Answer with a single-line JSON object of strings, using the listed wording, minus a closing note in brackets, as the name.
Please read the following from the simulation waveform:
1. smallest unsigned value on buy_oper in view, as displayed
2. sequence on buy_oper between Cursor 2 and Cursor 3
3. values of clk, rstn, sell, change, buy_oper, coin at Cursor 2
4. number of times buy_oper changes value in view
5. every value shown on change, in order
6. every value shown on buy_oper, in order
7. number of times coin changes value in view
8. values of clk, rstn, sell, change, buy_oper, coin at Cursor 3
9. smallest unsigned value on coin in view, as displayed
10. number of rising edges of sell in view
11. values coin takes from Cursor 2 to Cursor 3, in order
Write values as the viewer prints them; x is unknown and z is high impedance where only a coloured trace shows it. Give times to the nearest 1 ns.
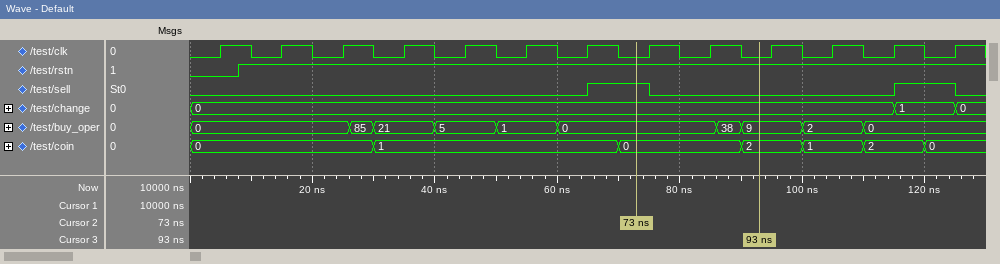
{"smallest unsigned value on buy_oper in view, as displayed": "0", "sequence on buy_oper between Cursor 2 and Cursor 3": "0, 38, 9", "values of clk, rstn, sell, change, buy_oper, coin at Cursor 2": "clk=0, rstn=1, sell=1, change=0, buy_oper=0, coin=0", "number of times buy_oper changes value in view": "9", "every value shown on change, in order": "0, 1, 0", "every value shown on buy_oper, in order": "0, 85, 21, 5, 1, 0, 38, 9, 2, 0", "number of times coin changes value in view": "6", "values of clk, rstn, sell, change, buy_oper, coin at Cursor 3": "clk=0, rstn=1, sell=0, change=0, buy_oper=9, coin=2", "smallest unsigned value on coin in view, as displayed": "0", "number of rising edges of sell in view": "2", "values coin takes from Cursor 2 to Cursor 3, in order": "0, 2"}
